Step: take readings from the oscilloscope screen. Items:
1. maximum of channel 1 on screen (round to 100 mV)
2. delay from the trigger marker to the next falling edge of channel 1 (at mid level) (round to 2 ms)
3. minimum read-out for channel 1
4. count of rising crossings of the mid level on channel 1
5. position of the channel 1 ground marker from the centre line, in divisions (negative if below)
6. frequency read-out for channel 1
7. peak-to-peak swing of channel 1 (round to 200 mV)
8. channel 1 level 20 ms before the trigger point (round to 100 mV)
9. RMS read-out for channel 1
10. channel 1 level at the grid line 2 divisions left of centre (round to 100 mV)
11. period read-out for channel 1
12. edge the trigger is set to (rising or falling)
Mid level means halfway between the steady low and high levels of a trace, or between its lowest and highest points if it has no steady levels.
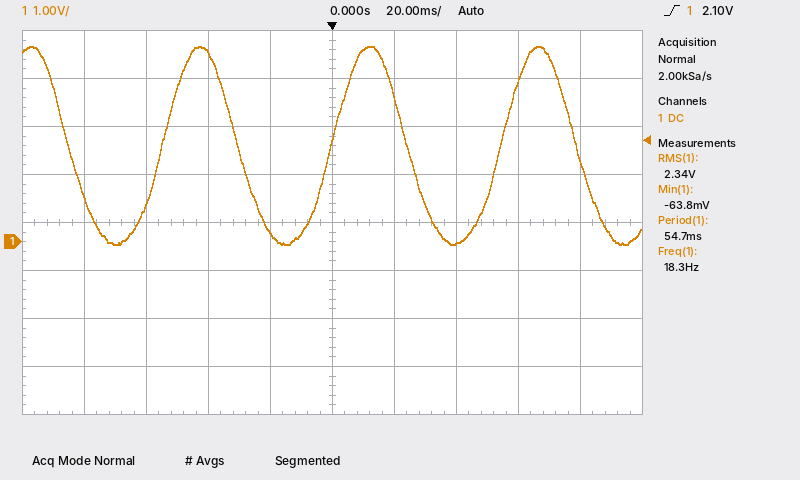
4.1 V
24 ms
-63.8 mV
3
-0.4 div
18.3 Hz
4.2 V
200 mV
2.34 V
3.9 V
54.7 ms
rising
